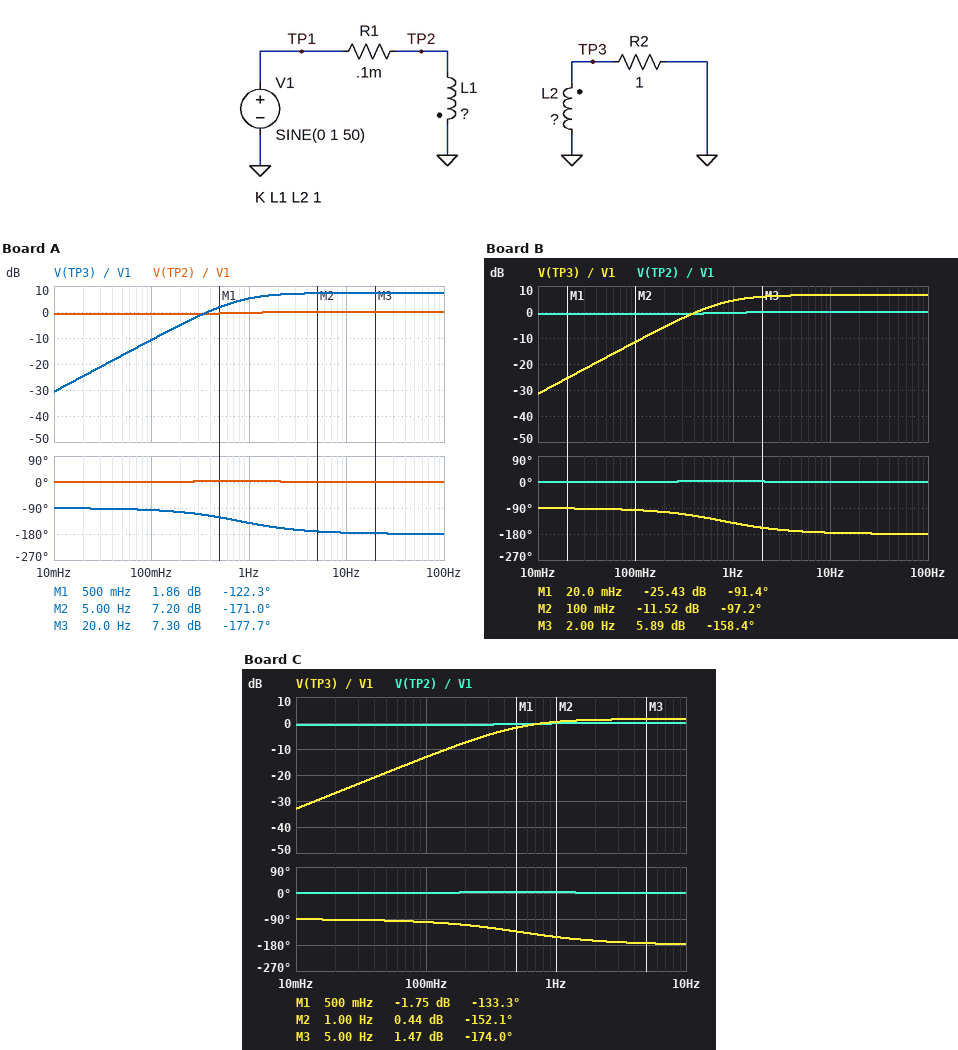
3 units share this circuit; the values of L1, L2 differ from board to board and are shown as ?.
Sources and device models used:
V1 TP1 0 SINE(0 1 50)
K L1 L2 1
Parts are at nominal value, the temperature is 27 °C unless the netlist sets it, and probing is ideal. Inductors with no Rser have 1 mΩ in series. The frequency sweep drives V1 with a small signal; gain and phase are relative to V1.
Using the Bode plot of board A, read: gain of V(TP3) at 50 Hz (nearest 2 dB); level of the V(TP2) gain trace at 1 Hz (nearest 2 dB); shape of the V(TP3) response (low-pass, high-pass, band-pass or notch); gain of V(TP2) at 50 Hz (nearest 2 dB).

8 dB
0 dB
high-pass
0 dB
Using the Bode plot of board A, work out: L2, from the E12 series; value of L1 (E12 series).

1.2 mH
220 µH
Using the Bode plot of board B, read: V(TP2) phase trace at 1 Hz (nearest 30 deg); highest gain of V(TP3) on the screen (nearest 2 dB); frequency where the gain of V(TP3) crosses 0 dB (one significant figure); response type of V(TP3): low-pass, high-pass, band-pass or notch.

0 deg
6 dB
400 mHz
high-pass
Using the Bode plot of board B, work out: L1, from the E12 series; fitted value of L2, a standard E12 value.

220 µH
1 mH
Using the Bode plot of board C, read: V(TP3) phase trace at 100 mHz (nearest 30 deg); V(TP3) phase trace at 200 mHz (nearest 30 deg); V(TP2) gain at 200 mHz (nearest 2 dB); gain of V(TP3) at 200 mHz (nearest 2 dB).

-90 deg
-120 deg
0 dB
-8 dB
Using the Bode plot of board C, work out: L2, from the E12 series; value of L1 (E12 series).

470 µH
330 µH
